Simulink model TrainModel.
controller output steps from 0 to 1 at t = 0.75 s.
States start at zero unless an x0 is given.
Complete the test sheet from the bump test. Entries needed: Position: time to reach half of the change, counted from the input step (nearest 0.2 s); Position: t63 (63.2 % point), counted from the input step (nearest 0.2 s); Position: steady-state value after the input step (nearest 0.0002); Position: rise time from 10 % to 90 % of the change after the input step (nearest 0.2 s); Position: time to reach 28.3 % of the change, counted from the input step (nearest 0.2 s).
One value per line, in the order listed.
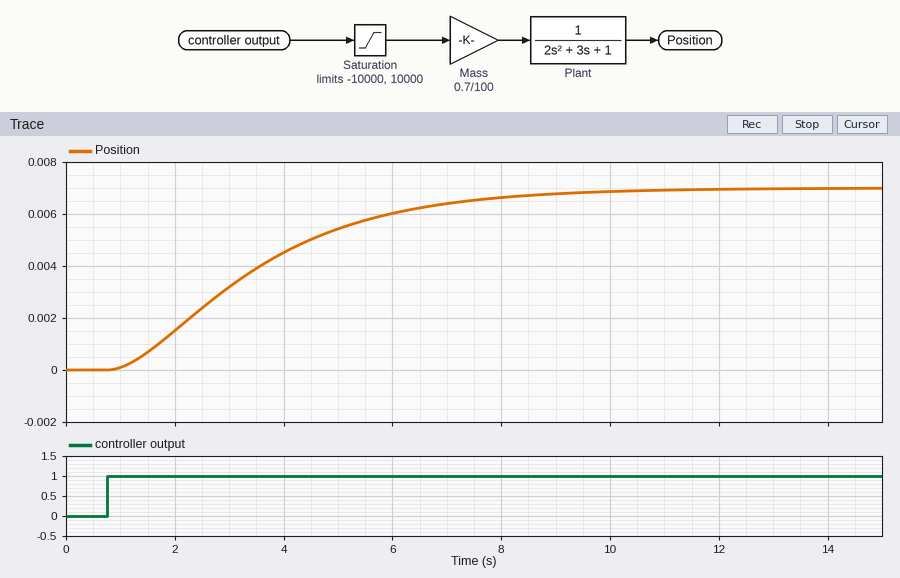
2.4 s
3.2 s
0.0070
5.2 s
1.6 s
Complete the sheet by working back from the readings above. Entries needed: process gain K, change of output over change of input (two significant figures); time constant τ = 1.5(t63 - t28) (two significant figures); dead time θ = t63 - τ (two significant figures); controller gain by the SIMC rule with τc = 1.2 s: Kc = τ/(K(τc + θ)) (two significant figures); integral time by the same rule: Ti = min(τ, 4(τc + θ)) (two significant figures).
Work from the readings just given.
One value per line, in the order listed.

0.0070
2.4 s
0.80 s
170
2.4 s
